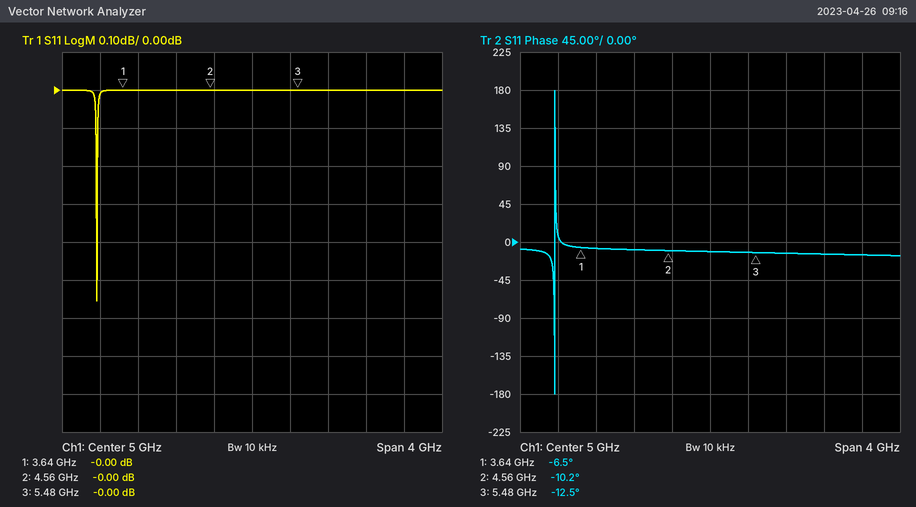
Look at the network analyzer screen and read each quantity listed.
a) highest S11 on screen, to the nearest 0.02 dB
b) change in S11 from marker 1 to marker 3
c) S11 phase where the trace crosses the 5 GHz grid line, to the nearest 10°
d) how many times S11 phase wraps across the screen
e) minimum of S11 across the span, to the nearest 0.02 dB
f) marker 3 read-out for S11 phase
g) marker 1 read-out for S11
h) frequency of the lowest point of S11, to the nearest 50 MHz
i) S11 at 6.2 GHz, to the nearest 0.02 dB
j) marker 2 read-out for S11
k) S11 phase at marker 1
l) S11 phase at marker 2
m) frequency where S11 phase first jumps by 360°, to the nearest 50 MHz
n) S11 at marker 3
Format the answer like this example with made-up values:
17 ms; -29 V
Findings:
0.00 dB; 0.00 dB; -10°; 1; -0.56 dB; -12.5°; -0.00 dB; 3.35 GHz; 0.00 dB; -0.00 dB; -6.5°; -10.2°; 3.35 GHz; -0.00 dB
